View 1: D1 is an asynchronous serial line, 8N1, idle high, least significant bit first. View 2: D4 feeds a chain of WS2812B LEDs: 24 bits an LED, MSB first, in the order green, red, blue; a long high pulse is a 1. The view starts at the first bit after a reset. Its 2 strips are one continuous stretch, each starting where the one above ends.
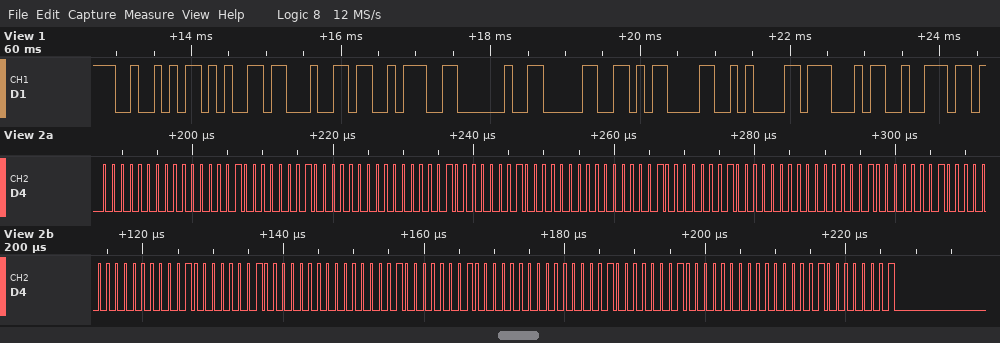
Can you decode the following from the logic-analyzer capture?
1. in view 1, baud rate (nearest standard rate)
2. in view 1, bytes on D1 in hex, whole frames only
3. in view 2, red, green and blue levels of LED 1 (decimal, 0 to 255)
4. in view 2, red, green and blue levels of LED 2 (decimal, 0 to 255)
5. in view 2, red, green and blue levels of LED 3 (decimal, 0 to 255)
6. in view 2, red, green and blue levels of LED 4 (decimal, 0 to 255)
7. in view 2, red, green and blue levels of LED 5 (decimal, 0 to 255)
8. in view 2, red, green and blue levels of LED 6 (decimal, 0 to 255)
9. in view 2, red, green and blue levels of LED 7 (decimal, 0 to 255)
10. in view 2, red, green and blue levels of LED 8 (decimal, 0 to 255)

9600 baud
0x52 0x65 0x64 0x3A 0x20 0x30 0x0D 0x0A 0x47 0x72
1, 0, 1
1, 0, 1
1, 0, 1
1, 0, 1
1, 0, 1
1, 0, 1
1, 0, 1
1, 0, 1
